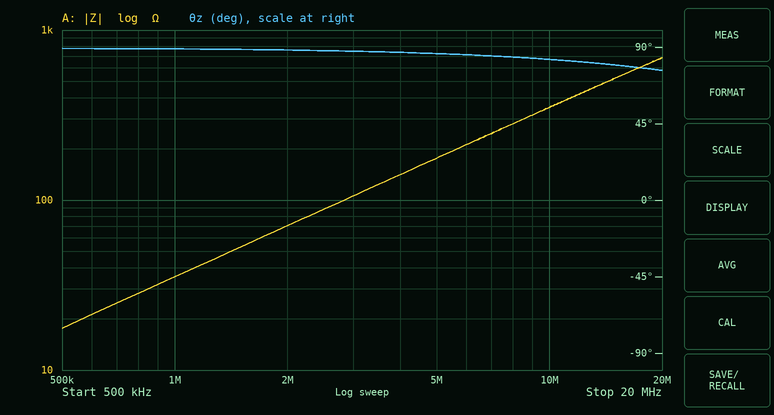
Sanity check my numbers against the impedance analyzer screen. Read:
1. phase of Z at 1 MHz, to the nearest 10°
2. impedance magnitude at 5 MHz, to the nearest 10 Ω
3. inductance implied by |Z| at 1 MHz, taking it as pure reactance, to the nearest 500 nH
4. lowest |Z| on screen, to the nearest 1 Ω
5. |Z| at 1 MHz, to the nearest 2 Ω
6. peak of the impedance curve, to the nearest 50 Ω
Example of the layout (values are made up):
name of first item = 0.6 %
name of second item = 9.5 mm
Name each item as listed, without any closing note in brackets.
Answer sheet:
phase of Z at 1 MHz, to the nearest 10° = 90°
impedance magnitude at 5 MHz, to the nearest 10 Ω = 180 Ω
inductance implied by |Z| at 1 MHz, taking it as pure reactance, to the nearest 500 nH = 5.5 µH
lowest |Z| on screen, to the nearest 1 Ω = 18 Ω
|Z| at 1 MHz, to the nearest 2 Ω = 36 Ω
peak of the impedance curve, to the nearest 50 Ω = 700 Ω
